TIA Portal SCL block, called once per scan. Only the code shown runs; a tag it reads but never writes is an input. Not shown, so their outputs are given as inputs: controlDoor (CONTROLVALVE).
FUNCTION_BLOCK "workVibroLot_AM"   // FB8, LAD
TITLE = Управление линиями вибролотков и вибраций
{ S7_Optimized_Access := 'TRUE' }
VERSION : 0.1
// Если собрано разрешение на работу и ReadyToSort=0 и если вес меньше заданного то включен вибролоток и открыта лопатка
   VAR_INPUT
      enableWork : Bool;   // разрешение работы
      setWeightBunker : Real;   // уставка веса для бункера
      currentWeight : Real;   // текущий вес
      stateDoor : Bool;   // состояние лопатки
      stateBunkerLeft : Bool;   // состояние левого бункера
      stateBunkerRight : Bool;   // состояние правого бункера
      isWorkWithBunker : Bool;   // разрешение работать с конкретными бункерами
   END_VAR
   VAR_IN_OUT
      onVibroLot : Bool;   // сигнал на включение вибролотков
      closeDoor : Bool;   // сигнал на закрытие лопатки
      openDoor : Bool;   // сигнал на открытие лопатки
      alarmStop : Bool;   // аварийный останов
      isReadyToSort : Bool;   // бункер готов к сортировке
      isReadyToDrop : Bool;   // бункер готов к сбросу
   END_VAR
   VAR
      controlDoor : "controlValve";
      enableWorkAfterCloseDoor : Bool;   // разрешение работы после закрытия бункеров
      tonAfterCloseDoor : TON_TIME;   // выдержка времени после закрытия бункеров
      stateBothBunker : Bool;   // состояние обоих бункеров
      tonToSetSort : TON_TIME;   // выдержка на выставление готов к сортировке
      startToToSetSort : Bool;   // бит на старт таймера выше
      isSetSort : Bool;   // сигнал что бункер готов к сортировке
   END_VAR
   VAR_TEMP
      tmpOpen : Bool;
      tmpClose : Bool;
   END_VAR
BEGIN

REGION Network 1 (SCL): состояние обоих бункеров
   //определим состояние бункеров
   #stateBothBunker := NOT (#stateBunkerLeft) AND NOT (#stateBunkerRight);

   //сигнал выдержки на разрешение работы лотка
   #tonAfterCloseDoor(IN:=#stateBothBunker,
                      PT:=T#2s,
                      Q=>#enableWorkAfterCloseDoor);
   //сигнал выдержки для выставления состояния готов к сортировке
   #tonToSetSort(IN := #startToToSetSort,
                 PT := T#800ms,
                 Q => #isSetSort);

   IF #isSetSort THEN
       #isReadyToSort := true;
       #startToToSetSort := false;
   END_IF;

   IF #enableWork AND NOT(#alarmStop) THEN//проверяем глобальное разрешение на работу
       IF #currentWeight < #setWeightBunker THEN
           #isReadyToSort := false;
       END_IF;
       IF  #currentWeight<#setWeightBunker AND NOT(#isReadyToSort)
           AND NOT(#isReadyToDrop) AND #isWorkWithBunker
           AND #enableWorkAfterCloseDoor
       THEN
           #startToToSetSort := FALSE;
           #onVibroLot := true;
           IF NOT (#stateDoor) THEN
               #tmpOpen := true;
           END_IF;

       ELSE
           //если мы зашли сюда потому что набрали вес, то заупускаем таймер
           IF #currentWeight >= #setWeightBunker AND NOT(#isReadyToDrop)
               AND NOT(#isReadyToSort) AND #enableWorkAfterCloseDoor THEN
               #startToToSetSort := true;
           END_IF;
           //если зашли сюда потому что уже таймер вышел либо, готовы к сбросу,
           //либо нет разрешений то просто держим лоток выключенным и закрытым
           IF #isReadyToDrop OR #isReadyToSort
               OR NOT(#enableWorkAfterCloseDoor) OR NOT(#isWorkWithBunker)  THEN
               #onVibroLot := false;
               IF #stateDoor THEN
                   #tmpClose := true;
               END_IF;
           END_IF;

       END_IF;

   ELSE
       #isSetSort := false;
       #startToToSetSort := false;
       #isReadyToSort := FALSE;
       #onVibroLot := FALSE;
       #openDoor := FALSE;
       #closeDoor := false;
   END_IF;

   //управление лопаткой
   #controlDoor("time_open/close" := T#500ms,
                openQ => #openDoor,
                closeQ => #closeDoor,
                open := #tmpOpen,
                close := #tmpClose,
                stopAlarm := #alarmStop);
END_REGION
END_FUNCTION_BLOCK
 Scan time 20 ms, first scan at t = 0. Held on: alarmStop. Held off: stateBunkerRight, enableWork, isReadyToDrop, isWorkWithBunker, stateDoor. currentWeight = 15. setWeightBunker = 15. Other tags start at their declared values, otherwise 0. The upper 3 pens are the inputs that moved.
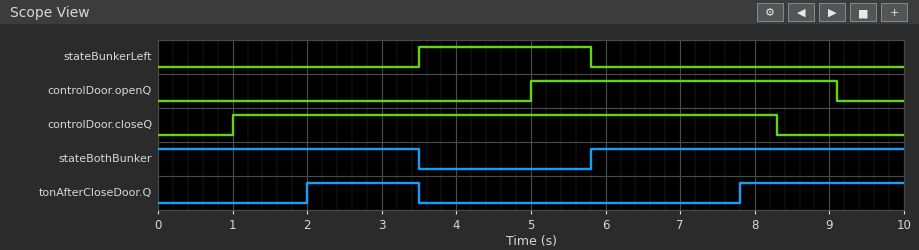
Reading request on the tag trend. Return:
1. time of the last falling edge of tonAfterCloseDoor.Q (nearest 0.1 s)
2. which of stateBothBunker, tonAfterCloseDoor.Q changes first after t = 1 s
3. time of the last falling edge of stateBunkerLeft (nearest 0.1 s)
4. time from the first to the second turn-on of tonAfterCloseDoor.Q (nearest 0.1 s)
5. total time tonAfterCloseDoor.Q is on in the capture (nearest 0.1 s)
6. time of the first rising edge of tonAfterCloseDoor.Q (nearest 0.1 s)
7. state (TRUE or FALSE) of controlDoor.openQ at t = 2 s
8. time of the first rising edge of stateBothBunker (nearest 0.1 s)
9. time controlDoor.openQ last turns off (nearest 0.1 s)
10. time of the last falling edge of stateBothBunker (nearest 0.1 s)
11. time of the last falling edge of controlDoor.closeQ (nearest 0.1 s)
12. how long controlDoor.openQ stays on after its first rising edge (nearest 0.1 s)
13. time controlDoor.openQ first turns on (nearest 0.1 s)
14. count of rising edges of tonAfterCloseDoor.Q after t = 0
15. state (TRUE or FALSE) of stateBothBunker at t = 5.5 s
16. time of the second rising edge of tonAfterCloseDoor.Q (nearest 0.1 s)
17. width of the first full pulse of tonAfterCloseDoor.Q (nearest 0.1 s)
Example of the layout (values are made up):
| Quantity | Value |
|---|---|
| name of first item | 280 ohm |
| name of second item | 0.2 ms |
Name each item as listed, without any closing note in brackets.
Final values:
| Quantity | Value |
|---|---|
| time of the last falling edge of tonAfterCloseDoor.Q | 3.5 s |
| which of stateBothBunker, tonAfterCloseDoor.Q changes first after t = 1 s | tonAfterCloseDoor.Q |
| time of the last falling edge of stateBunkerLeft | 5.8 s |
| time from the first to the second turn-on of tonAfterCloseDoor.Q | 5.8 s |
| total time tonAfterCloseDoor.Q is on in the capture | 3.7 s |
| time of the first rising edge of tonAfterCloseDoor.Q | 2.0 s |
| state (TRUE or FALSE) of controlDoor.openQ at t = 2 s | FALSE |
| time of the first rising edge of stateBothBunker | 5.8 s |
| time controlDoor.openQ last turns off | 9.1 s |
| time of the last falling edge of stateBothBunker | 3.5 s |
| time of the last falling edge of controlDoor.closeQ | 8.3 s |
| how long controlDoor.openQ stays on after its first rising edge | 4.1 s |
| time controlDoor.openQ first turns on | 5.0 s |
| count of rising edges of tonAfterCloseDoor.Q after t = 0 | 2 |
| state (TRUE or FALSE) of stateBothBunker at t = 5.5 s | FALSE |
| time of the second rising edge of tonAfterCloseDoor.Q | 7.8 s |
| width of the first full pulse of tonAfterCloseDoor.Q | 1.5 s |
